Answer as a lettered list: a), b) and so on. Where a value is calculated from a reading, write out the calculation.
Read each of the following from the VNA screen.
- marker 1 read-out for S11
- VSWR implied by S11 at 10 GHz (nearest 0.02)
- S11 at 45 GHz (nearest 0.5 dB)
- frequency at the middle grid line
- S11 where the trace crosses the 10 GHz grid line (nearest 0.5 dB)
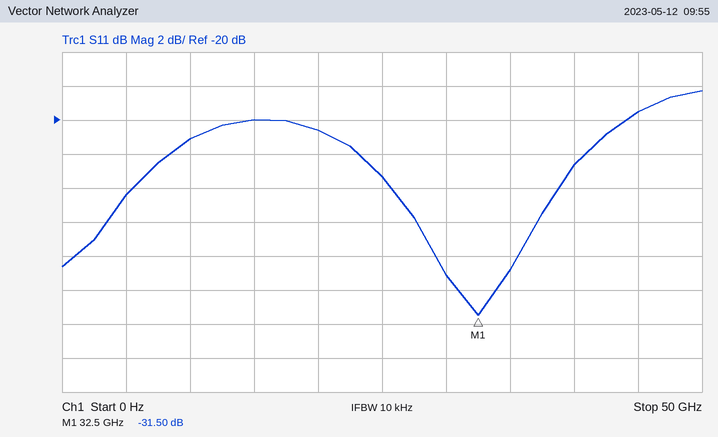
a) -31.50 dB
b) |Γ| = 10^(-21/20) = 0.0891; VSWR = (1 + 0.0891)/(1 − 0.0891) ≈ 1.20
c) -19.5 dB
d) 25 GHz
e) -21.0 dB
